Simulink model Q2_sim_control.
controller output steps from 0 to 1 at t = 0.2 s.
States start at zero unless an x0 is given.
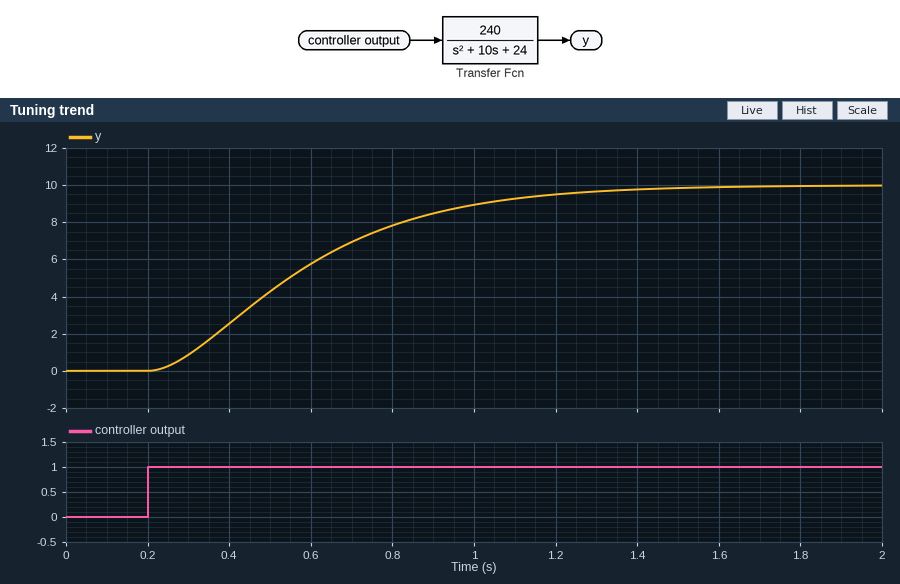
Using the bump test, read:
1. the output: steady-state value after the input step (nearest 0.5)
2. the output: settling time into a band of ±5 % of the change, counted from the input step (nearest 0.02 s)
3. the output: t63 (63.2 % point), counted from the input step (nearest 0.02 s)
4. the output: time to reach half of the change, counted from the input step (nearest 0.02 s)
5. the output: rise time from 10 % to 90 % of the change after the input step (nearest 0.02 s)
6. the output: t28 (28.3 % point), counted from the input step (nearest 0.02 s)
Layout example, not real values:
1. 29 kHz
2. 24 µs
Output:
1. 10.0
2. 1.00 s
3. 0.44 s
4. 0.34 s
5. 0.70 s
6. 0.22 s
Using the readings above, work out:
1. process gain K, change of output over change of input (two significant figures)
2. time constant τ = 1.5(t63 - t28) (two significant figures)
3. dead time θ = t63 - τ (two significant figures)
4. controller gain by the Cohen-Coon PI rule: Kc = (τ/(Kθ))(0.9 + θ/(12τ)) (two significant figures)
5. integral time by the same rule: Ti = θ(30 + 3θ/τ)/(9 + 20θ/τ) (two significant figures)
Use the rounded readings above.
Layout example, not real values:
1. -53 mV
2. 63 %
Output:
1. 10
2. 0.33 s
3. 0.11 s
4. 0.28
5. 0.22 s
